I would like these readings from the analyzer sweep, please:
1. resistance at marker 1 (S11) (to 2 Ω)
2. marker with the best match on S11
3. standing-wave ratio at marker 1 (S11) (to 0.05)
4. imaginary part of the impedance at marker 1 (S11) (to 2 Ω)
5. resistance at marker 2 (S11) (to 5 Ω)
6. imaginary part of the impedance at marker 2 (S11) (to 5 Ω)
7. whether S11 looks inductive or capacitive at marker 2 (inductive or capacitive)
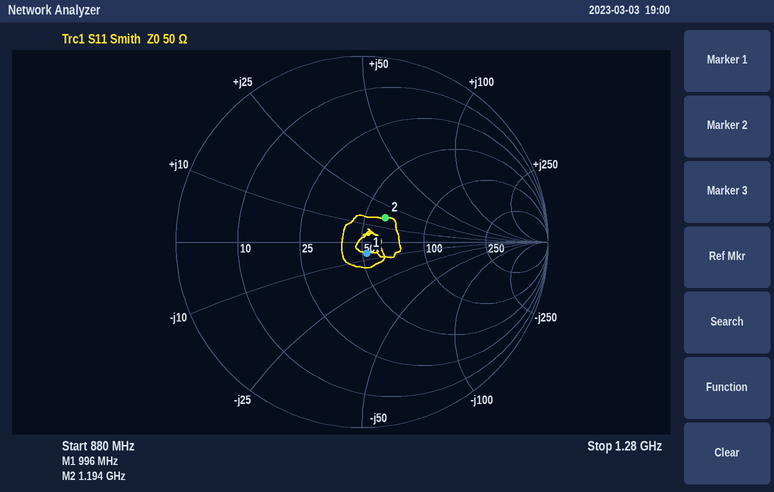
52 Ω
marker 1
1.15
-6 Ω
60 Ω
+15 Ω
inductive
